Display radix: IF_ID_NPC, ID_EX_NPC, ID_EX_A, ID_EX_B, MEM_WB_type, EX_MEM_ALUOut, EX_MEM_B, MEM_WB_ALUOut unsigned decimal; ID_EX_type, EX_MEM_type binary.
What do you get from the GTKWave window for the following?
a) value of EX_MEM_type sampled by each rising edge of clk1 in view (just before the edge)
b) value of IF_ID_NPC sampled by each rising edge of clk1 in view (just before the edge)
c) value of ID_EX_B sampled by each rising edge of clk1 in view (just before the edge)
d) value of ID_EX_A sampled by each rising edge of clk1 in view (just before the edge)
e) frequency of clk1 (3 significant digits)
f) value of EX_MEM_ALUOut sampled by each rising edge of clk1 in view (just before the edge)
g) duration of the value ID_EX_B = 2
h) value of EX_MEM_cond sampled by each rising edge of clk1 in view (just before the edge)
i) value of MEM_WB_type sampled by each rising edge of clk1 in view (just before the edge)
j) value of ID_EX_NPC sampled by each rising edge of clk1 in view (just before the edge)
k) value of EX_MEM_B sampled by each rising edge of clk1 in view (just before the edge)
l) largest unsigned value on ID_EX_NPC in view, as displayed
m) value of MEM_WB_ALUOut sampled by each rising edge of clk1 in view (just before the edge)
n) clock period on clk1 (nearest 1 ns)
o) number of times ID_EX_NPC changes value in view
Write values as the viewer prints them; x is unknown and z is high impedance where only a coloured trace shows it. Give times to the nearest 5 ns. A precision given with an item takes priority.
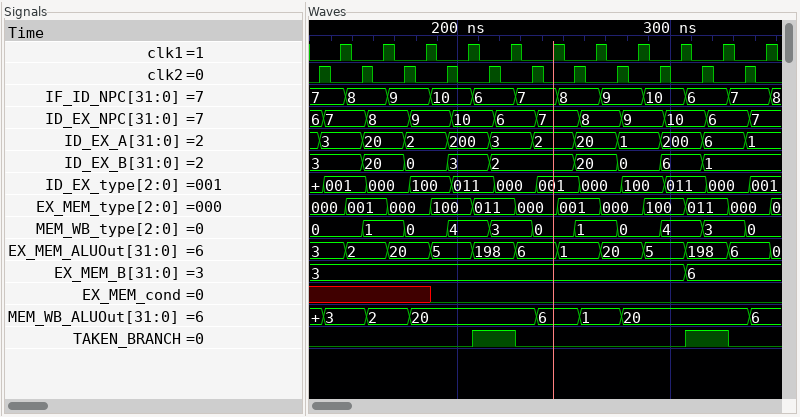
000, 001, 000, 100, 011, 000, 001, 000, 100, 011, 000
7, 8, 9, 10, 6, 7, 8, 9, 10, 6, 7
3, 20, 0, 3, 2, 2, 20, 0, 6, 1, 1
3, 20, 2, 200, 3, 2, 20, 1, 200, 6, 1
50.0 MHz
3, 2, 20, 5, 198, 6, 1, 20, 5, 198, 6
40 ns
x x x 0 0 0 0 0 0 0 0
0, 1, 0, 4, 3, 0, 1, 0, 4, 3, 0
7, 8, 9, 10, 6, 7, 8, 9, 10, 6, 7
3, 3, 3, 3, 3, 3, 3, 3, 3, 6, 6
10
3, 2, 20, 20, 20, 6, 1, 20, 20, 20, 6
20 ns
11
